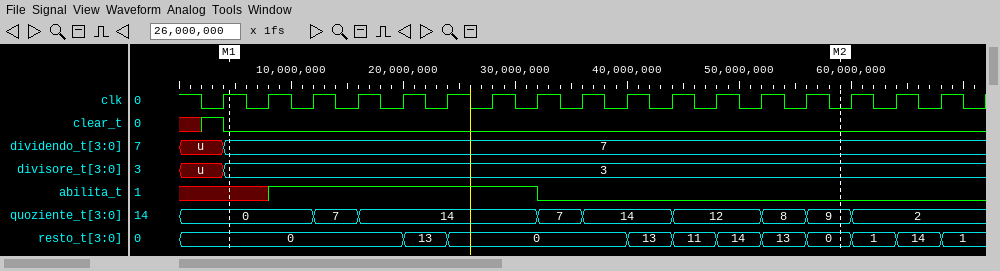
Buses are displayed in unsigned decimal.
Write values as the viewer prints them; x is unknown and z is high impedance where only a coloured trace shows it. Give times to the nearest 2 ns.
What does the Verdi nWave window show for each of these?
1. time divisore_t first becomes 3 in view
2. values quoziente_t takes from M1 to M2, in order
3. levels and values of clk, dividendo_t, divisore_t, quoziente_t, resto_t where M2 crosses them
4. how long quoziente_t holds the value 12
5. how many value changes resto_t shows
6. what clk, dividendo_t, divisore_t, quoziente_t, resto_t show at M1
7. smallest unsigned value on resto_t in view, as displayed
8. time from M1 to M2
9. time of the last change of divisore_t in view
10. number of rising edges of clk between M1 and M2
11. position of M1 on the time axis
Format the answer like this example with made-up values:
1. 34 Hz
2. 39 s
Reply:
1. 4 ns
2. 0, 7, 14, 7, 14, 12, 8, 9
3. clk=0, dividendo_t=7, divisore_t=3, quoziente_t=9, resto_t=0
4. 8 ns
5. 10
6. clk=1, dividendo_t=7, divisore_t=3, quoziente_t=0, resto_t=0
7. 0
8. 54 ns
9. 4 ns
10. 13
11. 4 ns
